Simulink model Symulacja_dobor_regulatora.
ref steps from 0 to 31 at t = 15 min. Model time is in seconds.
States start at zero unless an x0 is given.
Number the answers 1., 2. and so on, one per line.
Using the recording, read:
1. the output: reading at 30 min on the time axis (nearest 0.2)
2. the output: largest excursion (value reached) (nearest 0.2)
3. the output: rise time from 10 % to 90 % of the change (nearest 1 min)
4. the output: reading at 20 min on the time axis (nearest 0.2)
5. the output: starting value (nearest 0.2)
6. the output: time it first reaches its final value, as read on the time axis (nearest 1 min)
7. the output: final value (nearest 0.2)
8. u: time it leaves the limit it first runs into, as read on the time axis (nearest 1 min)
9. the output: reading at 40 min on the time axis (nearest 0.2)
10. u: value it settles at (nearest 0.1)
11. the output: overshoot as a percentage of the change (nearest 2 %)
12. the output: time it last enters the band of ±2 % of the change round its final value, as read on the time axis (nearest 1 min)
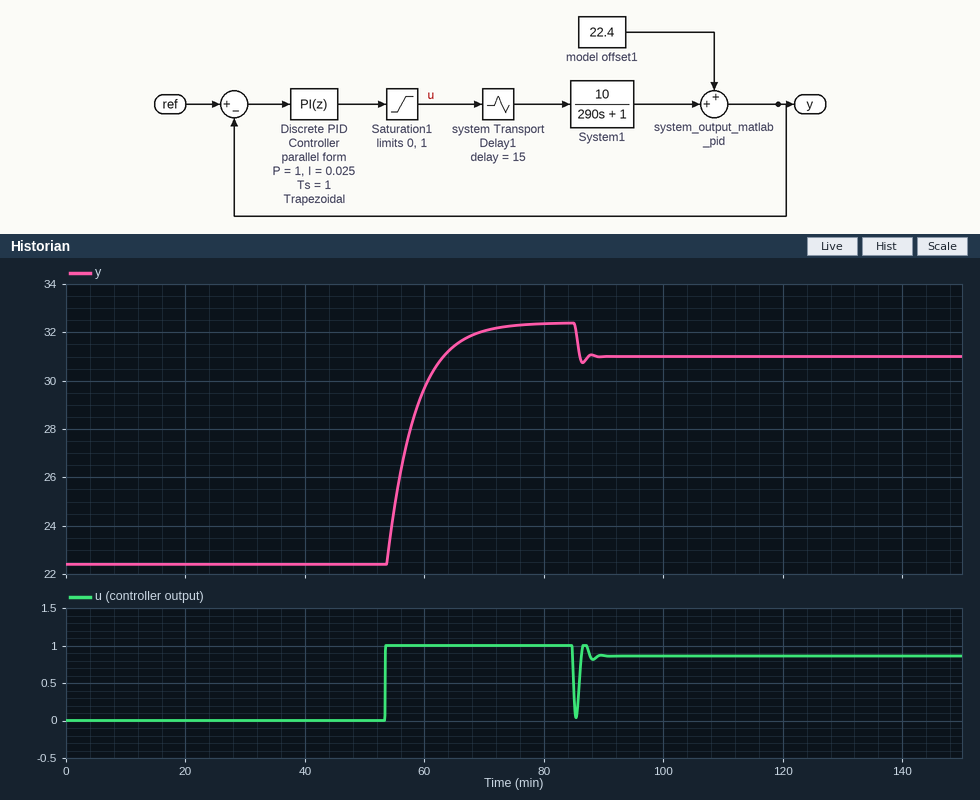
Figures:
1. 22.4
2. 32.4
3. 7 min
4. 22.4
5. 22.4
6. 63 min
7. 31.0
8. 53 min
9. 22.4
10. 0.9
11. 16 %
12. 87 min
